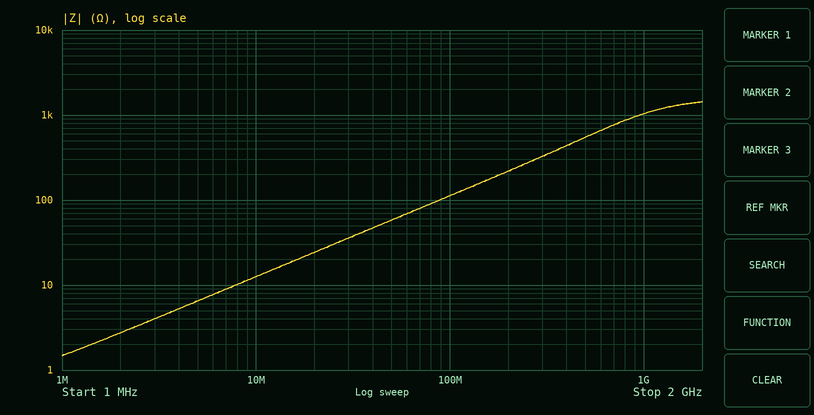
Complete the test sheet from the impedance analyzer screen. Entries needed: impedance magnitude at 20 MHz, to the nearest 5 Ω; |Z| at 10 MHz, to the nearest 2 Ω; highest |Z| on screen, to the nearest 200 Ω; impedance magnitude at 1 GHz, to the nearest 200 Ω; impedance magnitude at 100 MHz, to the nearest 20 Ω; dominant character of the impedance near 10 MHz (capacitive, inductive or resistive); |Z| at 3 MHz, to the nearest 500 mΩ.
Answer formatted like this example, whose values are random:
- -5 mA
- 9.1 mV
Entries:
- 25 Ω
- 12 Ω
- 1.4 kΩ
- 1.0 kΩ
- 120 Ω
- inductive
- 4.0 Ω
